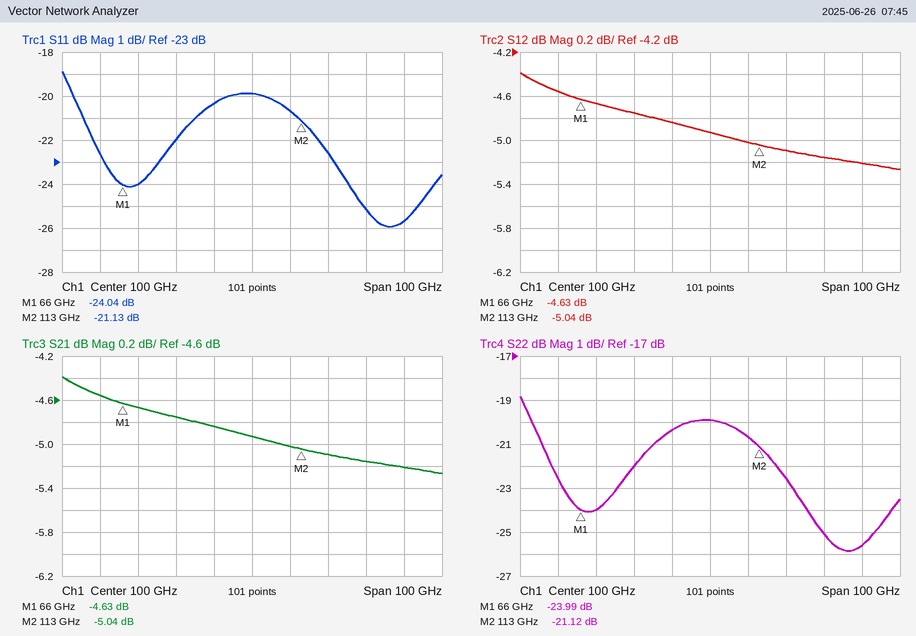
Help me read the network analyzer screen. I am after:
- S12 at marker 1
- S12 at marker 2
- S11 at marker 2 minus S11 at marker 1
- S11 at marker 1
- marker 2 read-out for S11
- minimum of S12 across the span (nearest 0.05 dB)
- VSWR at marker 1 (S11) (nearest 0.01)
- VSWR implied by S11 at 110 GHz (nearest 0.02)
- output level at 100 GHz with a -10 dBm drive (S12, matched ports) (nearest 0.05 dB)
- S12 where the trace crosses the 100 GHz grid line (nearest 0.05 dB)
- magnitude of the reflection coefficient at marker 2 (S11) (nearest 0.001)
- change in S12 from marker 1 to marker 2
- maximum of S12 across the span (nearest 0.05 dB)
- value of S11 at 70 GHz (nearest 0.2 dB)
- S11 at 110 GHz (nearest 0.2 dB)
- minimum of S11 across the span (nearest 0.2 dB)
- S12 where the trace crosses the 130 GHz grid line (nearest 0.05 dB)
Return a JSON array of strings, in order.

["-4.63 dB", "-5.04 dB", "2.91 dB", "-24.04 dB", "-21.13 dB", "-5.25 dB", "1.13", "1.20", "-14.95 dBm", "-4.95 dB", "0.088", "-0.41 dB", "-4.40 dB", "-24.0 dB", "-20.6 dB", "-26.0 dB", "-5.15 dB"]
